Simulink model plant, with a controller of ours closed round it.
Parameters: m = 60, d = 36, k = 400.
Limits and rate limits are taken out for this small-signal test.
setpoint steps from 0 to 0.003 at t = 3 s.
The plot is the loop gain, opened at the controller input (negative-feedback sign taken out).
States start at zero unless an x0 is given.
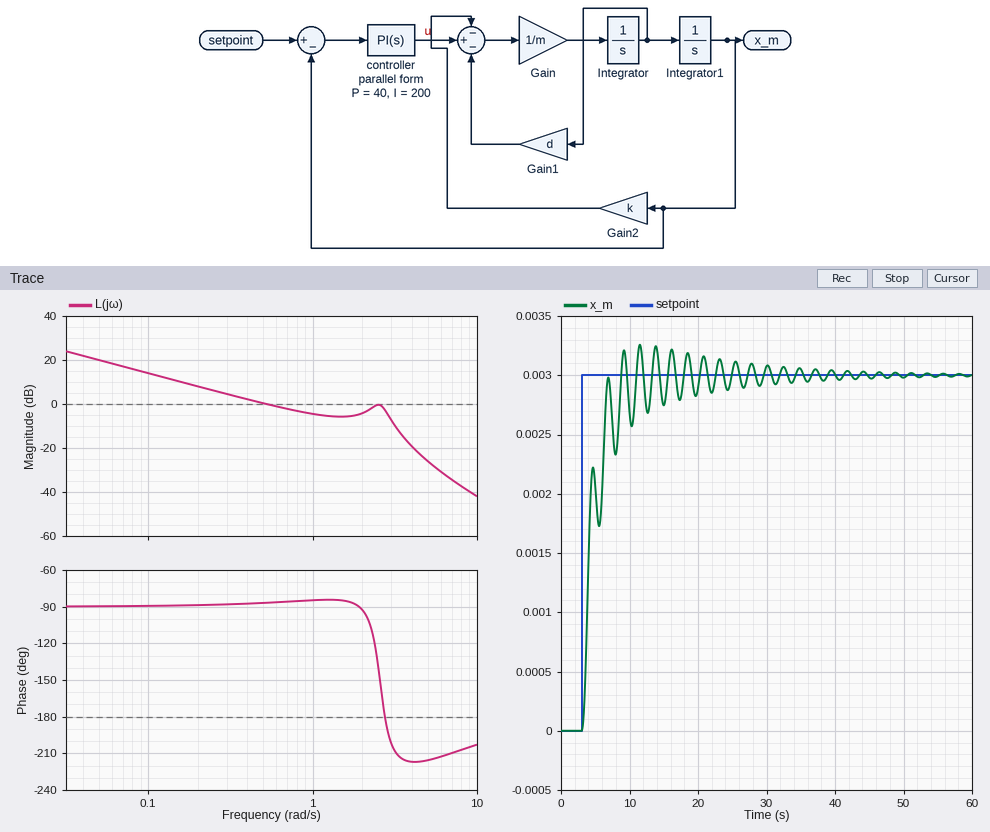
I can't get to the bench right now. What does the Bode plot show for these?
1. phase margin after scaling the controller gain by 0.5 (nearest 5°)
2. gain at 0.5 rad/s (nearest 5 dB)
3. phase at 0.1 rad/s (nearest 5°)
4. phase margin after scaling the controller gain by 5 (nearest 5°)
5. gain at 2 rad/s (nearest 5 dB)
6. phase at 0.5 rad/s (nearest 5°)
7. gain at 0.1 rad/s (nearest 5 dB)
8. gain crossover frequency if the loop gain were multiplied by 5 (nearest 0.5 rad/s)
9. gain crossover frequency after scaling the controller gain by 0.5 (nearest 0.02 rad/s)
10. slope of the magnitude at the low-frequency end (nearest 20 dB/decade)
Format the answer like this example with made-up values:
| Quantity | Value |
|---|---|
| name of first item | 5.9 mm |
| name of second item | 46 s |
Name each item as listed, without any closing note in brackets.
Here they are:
| Quantity | Value |
|---|---|
| phase margin after scaling the controller gain by 0.5 | 90° |
| gain at 0.5 rad/s | 0 dB |
| phase at 0.1 rad/s | -90° |
| phase margin after scaling the controller gain by 5 | -35° |
| gain at 2 rad/s | -5 dB |
| phase at 0.5 rad/s | -85° |
| gain at 0.1 rad/s | 15 dB |
| gain crossover frequency if the loop gain were multiplied by 5 | 3.5 rad/s |
| gain crossover frequency after scaling the controller gain by 0.5 | 0.26 rad/s |
| slope of the magnitude at the low-frequency end | -20 dB/decade |
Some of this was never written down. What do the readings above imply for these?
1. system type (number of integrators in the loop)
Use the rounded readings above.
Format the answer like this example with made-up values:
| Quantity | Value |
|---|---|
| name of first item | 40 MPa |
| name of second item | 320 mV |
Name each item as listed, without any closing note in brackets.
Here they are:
| Quantity | Value |
|---|---|
| system type | 1 |
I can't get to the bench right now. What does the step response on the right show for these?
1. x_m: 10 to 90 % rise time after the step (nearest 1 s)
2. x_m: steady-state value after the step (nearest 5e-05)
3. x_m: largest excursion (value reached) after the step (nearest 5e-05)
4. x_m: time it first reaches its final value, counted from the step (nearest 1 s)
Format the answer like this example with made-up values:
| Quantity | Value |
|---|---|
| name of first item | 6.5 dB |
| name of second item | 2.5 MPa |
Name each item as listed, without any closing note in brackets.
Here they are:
| Quantity | Value |
|---|---|
| x_m: 10 to 90 % rise time after the step | 3 s |
| x_m: steady-state value after the step | 0.00300 |
| x_m: largest excursion (value reached) after the step | 0.00325 |
| x_m: time it first reaches its final value, counted from the step | 6 s |
